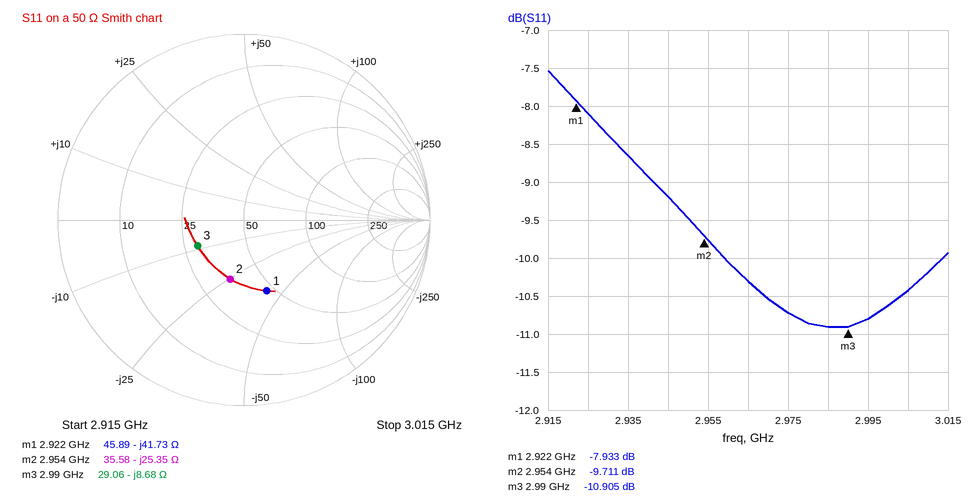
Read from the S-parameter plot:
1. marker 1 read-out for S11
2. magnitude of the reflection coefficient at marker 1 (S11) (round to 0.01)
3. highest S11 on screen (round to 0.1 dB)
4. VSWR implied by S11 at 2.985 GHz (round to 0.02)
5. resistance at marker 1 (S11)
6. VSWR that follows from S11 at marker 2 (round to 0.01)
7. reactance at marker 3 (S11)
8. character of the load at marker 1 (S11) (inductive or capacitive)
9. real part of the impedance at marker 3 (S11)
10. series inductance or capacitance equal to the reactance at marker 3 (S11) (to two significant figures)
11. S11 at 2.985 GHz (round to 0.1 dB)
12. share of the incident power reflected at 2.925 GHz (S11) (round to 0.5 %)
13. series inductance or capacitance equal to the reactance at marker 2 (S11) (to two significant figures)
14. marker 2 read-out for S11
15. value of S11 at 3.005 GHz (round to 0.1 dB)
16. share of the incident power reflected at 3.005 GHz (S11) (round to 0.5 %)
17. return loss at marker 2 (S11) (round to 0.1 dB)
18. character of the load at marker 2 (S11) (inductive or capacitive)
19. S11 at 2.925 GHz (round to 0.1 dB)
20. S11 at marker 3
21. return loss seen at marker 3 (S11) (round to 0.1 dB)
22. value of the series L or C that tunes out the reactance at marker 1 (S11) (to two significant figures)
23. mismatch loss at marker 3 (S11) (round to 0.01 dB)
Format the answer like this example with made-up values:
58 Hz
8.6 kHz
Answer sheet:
-7.933 dB
0.40
-7.5 dB
1.80
45.89 Ω
1.97
-8.68 Ω
capacitive
29.06 Ω
6.1 pF
-10.9 dB
15.5 %
2.1 pF
-9.711 dB
-10.4 dB
9.0 %
9.7 dB
capacitive
-8.1 dB
-10.905 dB
10.9 dB
2.3 nH
0.37 dB
